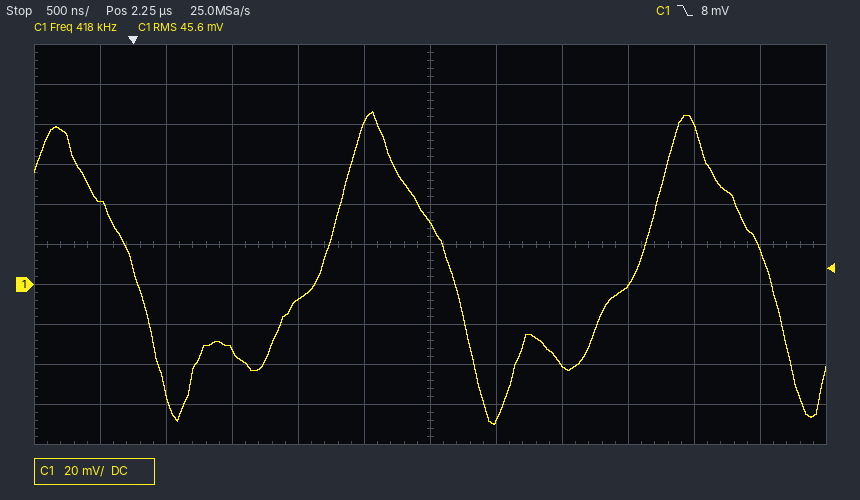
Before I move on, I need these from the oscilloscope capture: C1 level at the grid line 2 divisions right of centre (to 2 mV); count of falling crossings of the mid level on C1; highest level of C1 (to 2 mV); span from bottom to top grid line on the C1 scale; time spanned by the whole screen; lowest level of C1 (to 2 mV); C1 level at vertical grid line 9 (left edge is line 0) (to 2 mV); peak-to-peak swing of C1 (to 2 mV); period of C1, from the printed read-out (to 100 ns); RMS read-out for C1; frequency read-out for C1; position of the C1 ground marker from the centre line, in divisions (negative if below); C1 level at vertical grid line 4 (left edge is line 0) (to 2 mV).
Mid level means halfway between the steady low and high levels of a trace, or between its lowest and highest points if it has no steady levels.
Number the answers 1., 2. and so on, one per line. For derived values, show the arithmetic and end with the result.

1. -40 mV
2. 3
3. 86 mV
4. 200 mV
5. 6 µs
6. -70 mV
7. 0 mV
8. 86 mV − (-70 mV) = 156 mV
9. 1 / 418 kHz ≈ 2.4 µs
10. 45.6 mV
11. 418 kHz
12. -1.0 div
13. -8 mV
